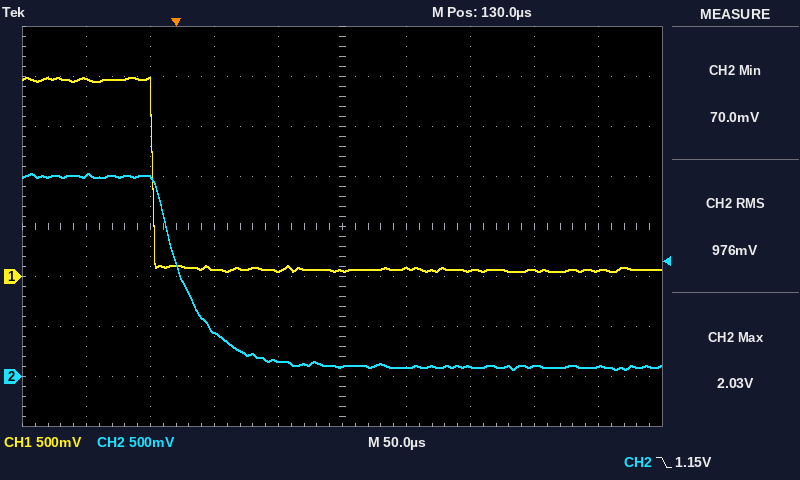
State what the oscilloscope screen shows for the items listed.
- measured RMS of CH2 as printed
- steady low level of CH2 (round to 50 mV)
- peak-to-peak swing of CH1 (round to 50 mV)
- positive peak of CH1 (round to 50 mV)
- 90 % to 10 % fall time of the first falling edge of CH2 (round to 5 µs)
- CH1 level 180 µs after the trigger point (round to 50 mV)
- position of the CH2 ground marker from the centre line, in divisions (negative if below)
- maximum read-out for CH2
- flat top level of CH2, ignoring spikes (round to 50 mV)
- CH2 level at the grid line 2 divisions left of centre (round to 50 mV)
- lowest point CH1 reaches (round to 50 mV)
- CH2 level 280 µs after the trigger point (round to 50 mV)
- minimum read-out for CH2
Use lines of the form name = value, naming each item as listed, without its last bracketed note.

measured RMS of CH2 as printed = 976 mV
steady low level of CH2 = 100 mV
peak-to-peak swing of CH1 = 1.95 V
positive peak of CH1 = 2.00 V
90 % to 10 % fall time of the first falling edge of CH2 = 60 µs
CH1 level 180 µs after the trigger point = 100 mV
position of the CH2 ground marker from the centre line, in divisions = -3.0 div
maximum read-out for CH2 = 2.03 V
flat top level of CH2, ignoring spikes = 2.00 V
CH2 level at the grid line 2 divisions left of centre = 450 mV
lowest point CH1 reaches = 50 mV
CH2 level 280 µs after the trigger point = 100 mV
minimum read-out for CH2 = 70.0 mV
